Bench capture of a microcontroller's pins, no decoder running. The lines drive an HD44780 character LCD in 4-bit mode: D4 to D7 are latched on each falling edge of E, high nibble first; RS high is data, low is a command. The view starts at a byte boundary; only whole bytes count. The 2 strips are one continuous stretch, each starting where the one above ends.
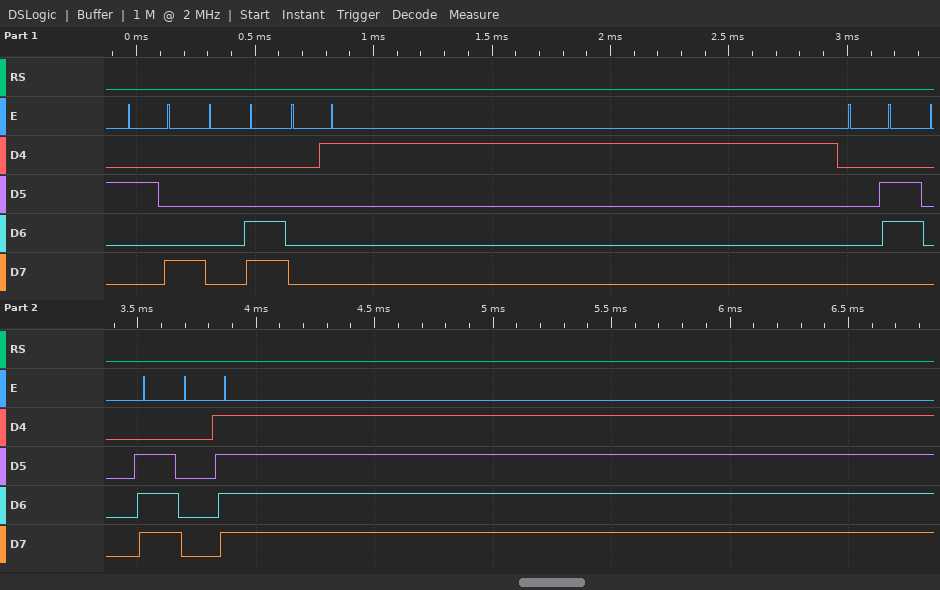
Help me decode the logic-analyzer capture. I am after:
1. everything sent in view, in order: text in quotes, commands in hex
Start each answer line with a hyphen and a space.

- 0x28 0x0C 0x01 0x06 0x0E 0x0F
